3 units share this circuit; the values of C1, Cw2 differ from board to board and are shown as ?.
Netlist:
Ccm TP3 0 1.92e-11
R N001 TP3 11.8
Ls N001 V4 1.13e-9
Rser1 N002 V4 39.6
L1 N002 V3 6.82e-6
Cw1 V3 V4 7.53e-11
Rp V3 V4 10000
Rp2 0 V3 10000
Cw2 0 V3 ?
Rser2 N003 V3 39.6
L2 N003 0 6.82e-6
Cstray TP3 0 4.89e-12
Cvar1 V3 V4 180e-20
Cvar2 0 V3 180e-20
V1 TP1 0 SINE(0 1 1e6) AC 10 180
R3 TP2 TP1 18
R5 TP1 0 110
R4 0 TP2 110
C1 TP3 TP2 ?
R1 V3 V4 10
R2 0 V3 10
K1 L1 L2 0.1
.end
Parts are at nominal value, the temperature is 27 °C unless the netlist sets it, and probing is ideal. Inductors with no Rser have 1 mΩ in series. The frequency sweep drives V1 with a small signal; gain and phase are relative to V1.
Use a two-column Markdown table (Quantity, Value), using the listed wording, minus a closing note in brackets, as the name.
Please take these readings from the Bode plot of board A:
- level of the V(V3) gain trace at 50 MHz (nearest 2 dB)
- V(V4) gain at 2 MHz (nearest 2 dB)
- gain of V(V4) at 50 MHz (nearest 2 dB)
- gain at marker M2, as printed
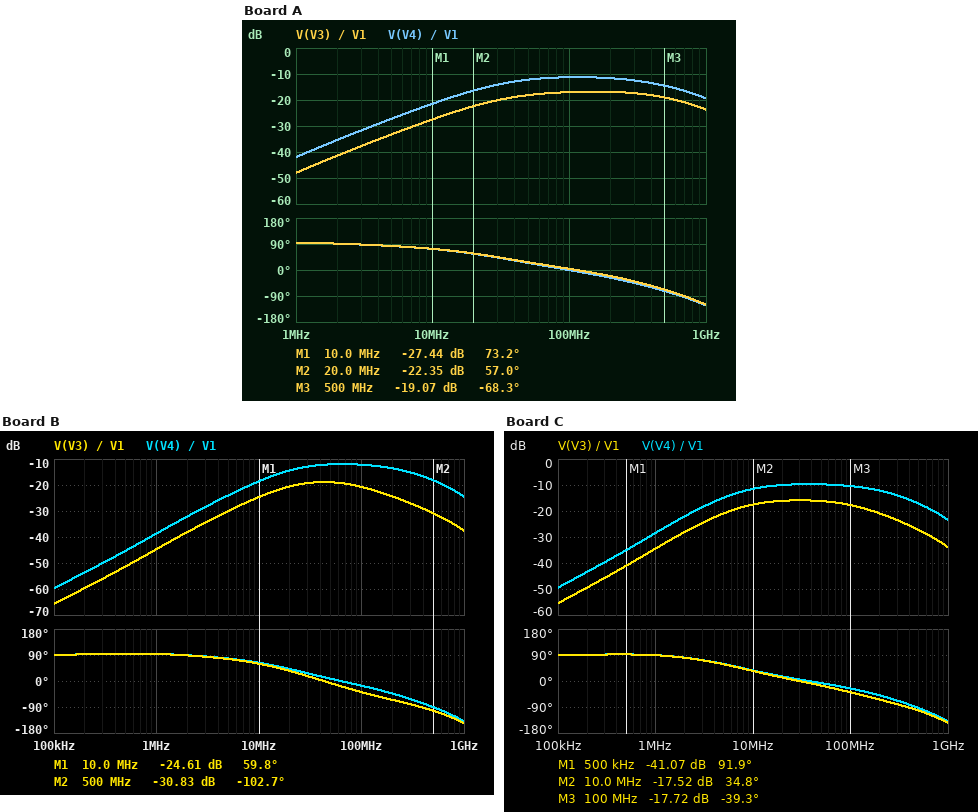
| Quantity | Value |
|---|---|
| level of the V(V3) gain trace at 50 MHz | -18 dB |
| V(V4) gain at 2 MHz | -36 dB |
| gain of V(V4) at 50 MHz | -12 dB |
| gain at marker M2, as printed | -22.35 dB |
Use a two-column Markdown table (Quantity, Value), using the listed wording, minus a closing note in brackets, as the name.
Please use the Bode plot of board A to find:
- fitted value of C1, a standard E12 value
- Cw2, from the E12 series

| Quantity | Value |
|---|---|
| fitted value of C1, a standard E12 value | 82 pF |
| Cw2, from the E12 series | 47 pF |
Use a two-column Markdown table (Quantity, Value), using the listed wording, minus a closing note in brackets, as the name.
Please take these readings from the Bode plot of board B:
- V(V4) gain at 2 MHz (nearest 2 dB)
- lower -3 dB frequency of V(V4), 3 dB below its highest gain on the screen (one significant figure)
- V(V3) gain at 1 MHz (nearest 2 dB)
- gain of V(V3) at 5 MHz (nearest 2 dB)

| Quantity | Value |
|---|---|
| V(V4) gain at 2 MHz | -32 dB |
| lower -3 dB frequency of V(V4), 3 dB below its highest gain on the screen | 20 MHz |
| V(V3) gain at 1 MHz | -44 dB |
| gain of V(V3) at 5 MHz | -30 dB |
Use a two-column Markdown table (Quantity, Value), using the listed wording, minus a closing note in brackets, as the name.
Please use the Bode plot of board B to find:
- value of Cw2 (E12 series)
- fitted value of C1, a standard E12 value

| Quantity | Value |
|---|---|
| value of Cw2 | 270 pF |
| fitted value of C1, a standard E12 value | 120 pF |
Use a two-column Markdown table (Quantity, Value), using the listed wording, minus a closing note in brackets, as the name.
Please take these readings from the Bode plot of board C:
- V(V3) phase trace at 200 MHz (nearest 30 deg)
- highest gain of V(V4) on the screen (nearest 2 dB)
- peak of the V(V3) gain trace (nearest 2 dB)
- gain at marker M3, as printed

| Quantity | Value |
|---|---|
| V(V3) phase trace at 200 MHz | -60 deg |
| highest gain of V(V4) on the screen | -10 dB |
| peak of the V(V3) gain trace | -16 dB |
| gain at marker M3, as printed | -17.72 dB |
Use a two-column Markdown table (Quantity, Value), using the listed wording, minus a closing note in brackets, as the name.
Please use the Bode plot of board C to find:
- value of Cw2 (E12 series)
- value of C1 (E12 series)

| Quantity | Value |
|---|---|
| value of Cw2 | 180 pF |
| value of C1 | 390 pF |
